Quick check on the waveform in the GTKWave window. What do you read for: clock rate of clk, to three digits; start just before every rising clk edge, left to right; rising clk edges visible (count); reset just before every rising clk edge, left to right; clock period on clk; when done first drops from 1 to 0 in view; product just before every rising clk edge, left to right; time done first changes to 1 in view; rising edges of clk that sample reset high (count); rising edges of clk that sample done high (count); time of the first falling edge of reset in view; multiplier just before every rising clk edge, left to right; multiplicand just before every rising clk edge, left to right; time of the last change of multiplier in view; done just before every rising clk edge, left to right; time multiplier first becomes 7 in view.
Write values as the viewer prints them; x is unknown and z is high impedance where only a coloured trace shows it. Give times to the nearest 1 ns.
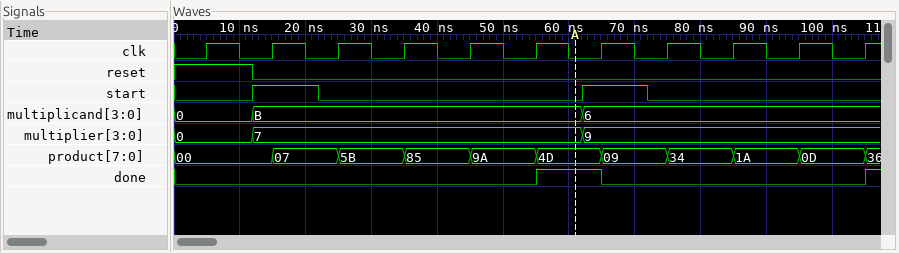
100 MHz
0 1 0 0 0 0 1 0 0 0 0
11
1 0 0 0 0 0 0 0 0 0 0
10 ns
65 ns
00, 00, 07, 5B, 85, 9A, 4D, 09, 34, 1A, 0D
55 ns
1
1
12 ns
0, 7, 7, 7, 7, 7, 9, 9, 9, 9, 9
0, B, B, B, B, B, 6, 6, 6, 6, 6
62 ns
0 0 0 0 0 0 1 0 0 0 0
12 ns
